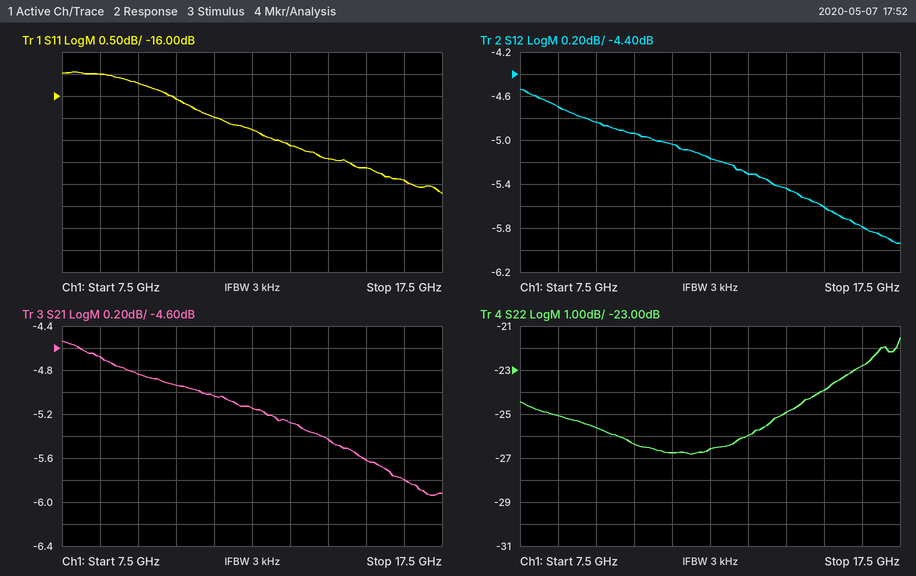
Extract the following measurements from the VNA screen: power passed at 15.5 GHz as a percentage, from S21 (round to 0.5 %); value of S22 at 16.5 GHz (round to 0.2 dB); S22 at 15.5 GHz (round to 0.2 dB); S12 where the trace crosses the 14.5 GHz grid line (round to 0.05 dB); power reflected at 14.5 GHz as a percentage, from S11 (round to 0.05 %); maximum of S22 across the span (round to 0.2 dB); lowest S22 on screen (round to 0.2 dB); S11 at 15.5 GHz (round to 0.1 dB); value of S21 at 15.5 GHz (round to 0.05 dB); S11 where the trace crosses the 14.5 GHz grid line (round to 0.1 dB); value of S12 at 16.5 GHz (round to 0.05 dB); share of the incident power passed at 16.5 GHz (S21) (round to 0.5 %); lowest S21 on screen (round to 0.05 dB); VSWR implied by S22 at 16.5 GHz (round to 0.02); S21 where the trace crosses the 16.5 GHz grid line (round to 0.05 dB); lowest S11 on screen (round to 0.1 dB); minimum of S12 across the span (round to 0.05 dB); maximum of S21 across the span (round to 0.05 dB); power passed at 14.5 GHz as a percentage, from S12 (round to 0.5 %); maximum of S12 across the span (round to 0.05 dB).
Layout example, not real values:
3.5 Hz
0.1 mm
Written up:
27.5 %
-22.8 dB
-24.0 dB
-5.45 dB
1.80 %
-21.6 dB
-26.8 dB
-17.6 dB
-5.60 dB
-17.4 dB
-5.80 dB
26.5 %
-5.95 dB
1.16
-5.80 dB
-18.2 dB
-5.95 dB
-4.55 dB
28.5 %
-4.55 dB
